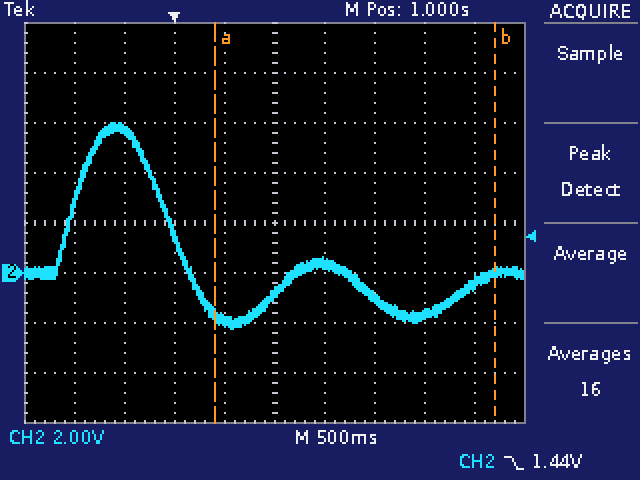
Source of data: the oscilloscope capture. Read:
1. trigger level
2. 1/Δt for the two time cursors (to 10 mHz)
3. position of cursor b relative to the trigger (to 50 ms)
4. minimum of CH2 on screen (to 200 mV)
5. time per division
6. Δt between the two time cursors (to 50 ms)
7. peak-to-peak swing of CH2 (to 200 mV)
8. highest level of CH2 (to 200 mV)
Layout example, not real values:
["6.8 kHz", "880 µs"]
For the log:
["1.44 V", "360 mHz", "+3.20 s", "-2.2 V", "500 ms", "2.80 s", "8.2 V", "6.0 V"]
